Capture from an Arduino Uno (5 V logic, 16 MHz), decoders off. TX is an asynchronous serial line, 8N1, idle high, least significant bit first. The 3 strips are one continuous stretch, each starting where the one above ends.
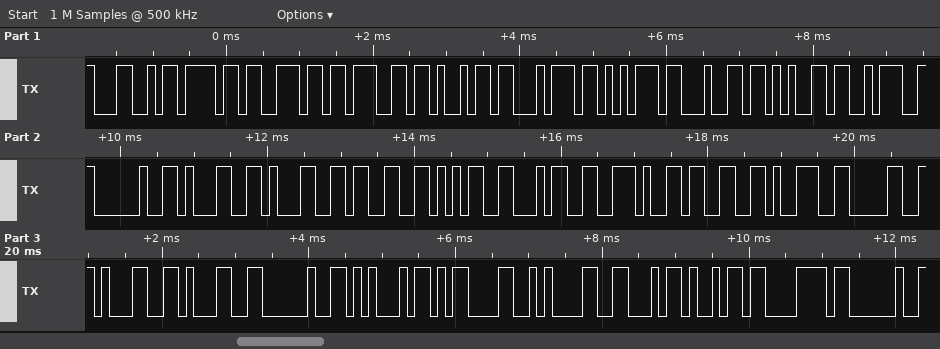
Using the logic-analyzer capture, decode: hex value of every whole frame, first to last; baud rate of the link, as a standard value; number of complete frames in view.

0x4C 0x6F 0x6E 0x67 0x69 0x74 0x75 0x64 0x65 0x3A 0x20 0x31 0x31 0x33 0x35 0x34 0x2E 0x33 0x39 0x30 0x31 0x31 0x20 0x45 0x0D 0x0A 0x46 0x69 0x78 0x20
9600 baud
30
